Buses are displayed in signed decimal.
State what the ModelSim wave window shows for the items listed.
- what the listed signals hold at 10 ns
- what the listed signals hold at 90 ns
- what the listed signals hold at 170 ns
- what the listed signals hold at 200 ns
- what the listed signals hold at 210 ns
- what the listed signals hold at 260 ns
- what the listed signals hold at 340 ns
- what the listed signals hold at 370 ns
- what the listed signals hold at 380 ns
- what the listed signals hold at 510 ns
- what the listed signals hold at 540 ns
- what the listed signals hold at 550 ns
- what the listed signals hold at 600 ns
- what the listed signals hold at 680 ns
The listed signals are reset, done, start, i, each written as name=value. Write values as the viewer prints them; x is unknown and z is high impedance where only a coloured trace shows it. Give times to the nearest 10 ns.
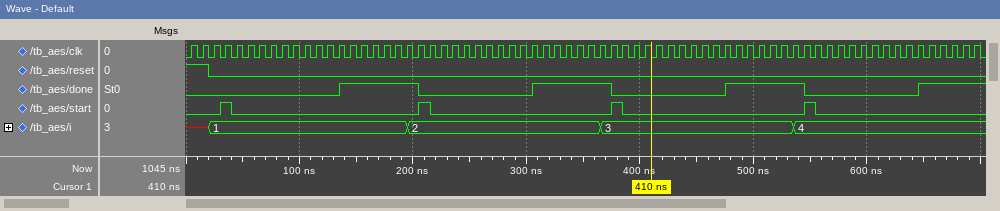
reset=1, done=0, start=0, i=x
reset=0, done=0, start=0, i=1
reset=0, done=1, start=0, i=1
reset=0, done=1, start=0, i=2
reset=0, done=0, start=1, i=2
reset=0, done=0, start=0, i=2
reset=0, done=1, start=0, i=2
reset=0, done=1, start=0, i=3
reset=0, done=0, start=1, i=3
reset=0, done=1, start=0, i=3
reset=0, done=1, start=0, i=4
reset=0, done=0, start=1, i=4
reset=0, done=0, start=0, i=4
reset=0, done=1, start=0, i=4
